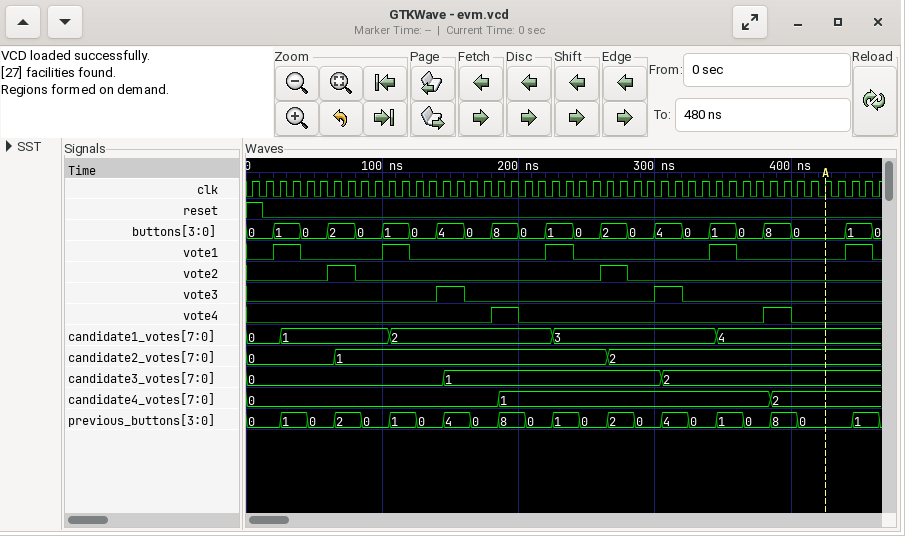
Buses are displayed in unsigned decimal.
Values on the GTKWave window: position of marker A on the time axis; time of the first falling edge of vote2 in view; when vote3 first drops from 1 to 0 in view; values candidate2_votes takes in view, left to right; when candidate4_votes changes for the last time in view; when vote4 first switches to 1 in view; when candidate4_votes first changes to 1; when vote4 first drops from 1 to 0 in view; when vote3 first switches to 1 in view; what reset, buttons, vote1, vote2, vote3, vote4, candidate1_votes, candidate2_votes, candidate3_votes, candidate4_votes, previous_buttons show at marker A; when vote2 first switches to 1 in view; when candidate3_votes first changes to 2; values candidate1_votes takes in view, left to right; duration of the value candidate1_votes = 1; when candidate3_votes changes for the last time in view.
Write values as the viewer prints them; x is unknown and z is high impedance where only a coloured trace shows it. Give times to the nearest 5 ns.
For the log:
425 ns
80 ns
160 ns
0, 1, 2
385 ns
180 ns
185 ns
200 ns
140 ns
reset=0, buttons=0, vote1=0, vote2=0, vote3=0, vote4=0, candidate1_votes=4, candidate2_votes=2, candidate3_votes=2, candidate4_votes=2, previous_buttons=0
60 ns
305 ns
0, 1, 2, 3, 4
80 ns
305 ns
